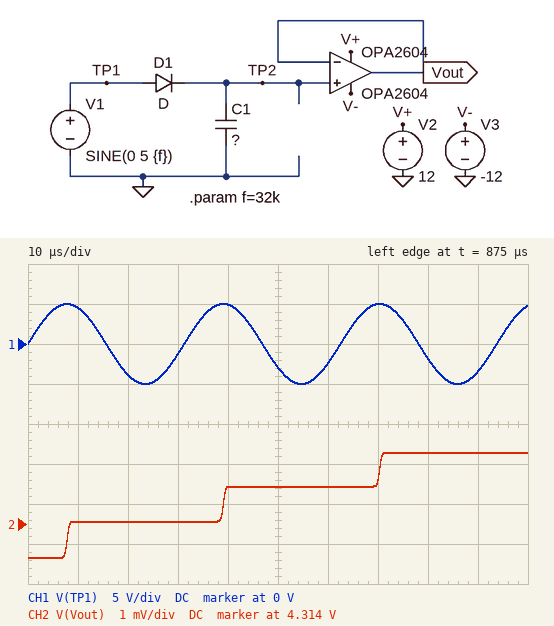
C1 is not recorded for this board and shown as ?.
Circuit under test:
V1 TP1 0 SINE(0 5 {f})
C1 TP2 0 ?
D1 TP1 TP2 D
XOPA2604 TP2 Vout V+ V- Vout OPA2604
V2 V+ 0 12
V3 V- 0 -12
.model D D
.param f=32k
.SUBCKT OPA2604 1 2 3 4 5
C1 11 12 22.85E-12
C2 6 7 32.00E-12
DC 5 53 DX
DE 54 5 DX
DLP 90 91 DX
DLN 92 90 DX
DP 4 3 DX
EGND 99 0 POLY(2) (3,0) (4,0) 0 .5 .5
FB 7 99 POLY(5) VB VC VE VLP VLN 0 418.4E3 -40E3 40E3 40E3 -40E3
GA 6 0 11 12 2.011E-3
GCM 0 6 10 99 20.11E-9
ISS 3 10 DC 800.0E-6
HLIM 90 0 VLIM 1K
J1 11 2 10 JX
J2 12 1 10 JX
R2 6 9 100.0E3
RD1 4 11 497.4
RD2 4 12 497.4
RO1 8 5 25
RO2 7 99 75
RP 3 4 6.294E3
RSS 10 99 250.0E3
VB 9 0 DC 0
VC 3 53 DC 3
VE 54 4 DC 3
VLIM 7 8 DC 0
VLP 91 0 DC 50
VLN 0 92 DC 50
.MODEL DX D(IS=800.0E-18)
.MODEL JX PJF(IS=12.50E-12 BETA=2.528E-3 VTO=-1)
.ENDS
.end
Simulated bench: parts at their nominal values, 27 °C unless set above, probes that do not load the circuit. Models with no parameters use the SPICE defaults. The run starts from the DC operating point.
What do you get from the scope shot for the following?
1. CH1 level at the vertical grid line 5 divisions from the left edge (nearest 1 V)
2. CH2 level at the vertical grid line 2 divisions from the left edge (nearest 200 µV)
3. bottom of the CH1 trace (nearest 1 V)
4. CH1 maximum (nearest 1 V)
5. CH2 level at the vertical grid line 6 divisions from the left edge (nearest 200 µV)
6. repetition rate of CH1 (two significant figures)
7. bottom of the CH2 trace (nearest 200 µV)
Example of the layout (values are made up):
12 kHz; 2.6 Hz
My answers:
-3 V; 4.3140 V; -5 V; 5 V; 4.3150 V; 32 kHz; 4.3132 V
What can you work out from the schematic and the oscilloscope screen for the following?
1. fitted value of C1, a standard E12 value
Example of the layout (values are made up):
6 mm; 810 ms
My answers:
3.3 µF
